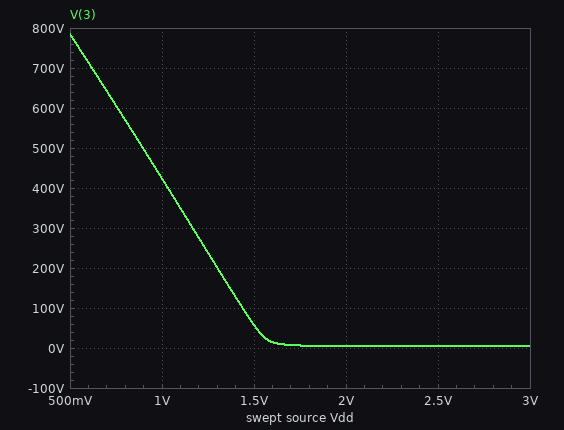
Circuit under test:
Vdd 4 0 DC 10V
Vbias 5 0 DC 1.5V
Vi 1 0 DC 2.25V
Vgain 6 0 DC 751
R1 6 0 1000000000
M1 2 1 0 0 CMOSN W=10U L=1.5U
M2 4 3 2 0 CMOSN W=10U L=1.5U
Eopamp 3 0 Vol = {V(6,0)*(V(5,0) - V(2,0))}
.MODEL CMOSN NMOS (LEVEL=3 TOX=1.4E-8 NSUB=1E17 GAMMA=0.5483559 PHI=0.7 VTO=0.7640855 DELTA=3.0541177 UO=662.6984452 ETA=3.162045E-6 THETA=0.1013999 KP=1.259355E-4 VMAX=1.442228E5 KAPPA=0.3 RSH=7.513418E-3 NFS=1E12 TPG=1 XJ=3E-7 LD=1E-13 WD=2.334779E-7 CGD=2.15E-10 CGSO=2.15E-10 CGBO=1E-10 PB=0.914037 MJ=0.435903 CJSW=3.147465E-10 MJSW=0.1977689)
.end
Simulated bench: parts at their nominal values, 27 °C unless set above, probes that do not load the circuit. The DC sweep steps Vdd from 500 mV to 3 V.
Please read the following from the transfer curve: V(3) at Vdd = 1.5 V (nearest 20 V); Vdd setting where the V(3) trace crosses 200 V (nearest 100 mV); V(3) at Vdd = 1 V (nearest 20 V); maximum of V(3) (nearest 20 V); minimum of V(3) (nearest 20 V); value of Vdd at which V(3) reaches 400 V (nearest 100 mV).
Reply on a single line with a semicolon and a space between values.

60 V; 1.3 V; 420 V; 780 V; 0 V; 1.0 V
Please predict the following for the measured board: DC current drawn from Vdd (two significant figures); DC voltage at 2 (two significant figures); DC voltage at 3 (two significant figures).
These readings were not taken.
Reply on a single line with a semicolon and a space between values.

510 µA; 1.5 V; 4.0 V
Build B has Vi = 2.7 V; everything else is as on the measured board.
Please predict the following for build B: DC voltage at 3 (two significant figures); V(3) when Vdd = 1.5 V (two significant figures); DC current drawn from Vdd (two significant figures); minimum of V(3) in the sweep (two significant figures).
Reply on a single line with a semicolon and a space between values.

4.4 V; 83 V; 780 µA; 4.5 V
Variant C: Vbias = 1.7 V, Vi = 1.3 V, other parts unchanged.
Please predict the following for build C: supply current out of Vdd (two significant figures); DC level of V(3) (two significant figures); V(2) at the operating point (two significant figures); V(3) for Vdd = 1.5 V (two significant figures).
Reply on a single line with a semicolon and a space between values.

88 µA; 3.3 V; 1.7 V; 160 V
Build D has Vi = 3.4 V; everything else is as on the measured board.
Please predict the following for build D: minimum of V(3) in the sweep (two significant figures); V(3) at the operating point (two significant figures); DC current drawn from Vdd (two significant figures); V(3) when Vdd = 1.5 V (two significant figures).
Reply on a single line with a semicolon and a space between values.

5.2 V; 5.0 V; 1.2 mA; 120 V
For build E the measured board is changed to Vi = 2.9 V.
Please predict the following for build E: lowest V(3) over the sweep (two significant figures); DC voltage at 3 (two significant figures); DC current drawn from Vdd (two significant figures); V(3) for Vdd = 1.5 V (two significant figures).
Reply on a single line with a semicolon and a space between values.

4.7 V; 4.5 V; 910 µA; 95 V
